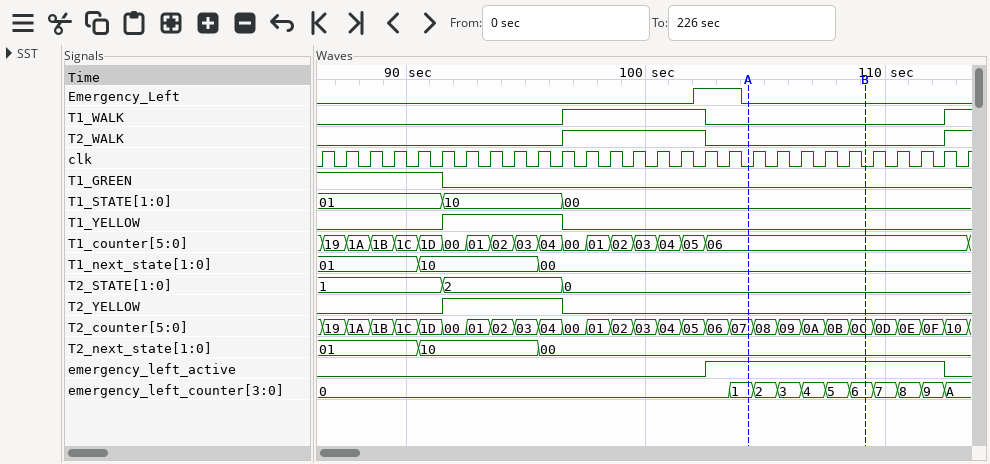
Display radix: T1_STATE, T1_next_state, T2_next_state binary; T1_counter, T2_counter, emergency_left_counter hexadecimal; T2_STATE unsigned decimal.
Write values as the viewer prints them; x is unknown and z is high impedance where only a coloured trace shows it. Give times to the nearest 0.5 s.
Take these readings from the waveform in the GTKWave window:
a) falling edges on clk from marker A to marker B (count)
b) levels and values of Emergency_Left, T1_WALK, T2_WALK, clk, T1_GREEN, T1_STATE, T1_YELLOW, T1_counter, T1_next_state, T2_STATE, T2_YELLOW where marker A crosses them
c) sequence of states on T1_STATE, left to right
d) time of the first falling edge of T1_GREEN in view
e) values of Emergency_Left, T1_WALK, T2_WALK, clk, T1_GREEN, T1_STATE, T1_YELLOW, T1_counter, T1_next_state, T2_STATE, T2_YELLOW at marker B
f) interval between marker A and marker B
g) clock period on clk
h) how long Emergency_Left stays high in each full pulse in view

5
Emergency_Left=0, T1_WALK=0, T2_WALK=0, clk=0, T1_GREEN=0, T1_STATE=00, T1_YELLOW=0, T1_counter=06, T1_next_state=00, T2_STATE=0, T2_YELLOW=0
01, 10, 00
91.5 s
Emergency_Left=0, T1_WALK=0, T2_WALK=0, clk=0, T1_GREEN=0, T1_STATE=00, T1_YELLOW=0, T1_counter=06, T1_next_state=00, T2_STATE=0, T2_YELLOW=0
5 s
1 s
2 s
